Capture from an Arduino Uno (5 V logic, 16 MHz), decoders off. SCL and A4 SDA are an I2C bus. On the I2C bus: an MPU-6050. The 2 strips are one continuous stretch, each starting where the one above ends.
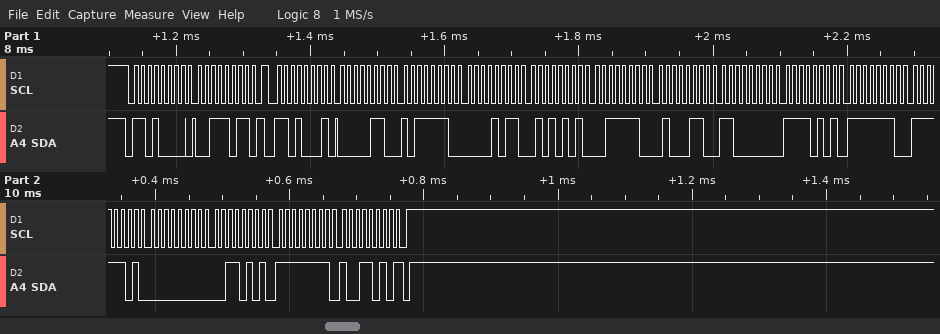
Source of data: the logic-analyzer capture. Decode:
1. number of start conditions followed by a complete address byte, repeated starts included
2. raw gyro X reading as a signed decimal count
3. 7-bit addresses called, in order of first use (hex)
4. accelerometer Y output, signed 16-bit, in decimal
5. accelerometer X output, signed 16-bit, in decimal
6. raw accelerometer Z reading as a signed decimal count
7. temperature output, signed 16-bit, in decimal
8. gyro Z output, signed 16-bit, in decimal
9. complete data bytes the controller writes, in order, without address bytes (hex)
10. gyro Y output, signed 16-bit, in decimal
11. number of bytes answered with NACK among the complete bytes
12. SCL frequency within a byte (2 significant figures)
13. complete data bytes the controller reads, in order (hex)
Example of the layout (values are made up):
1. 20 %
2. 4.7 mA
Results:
1. 2
2. -259
3. 0x68
4. 2901
5. 1726
6. 15942
7. -16139
8. -102
9. 3B
10. 53
11. 1
12. 100 kHz
13. 06 BE 0B 55 3E 46 C0 F5 FE FD 00 35 FF 9A
